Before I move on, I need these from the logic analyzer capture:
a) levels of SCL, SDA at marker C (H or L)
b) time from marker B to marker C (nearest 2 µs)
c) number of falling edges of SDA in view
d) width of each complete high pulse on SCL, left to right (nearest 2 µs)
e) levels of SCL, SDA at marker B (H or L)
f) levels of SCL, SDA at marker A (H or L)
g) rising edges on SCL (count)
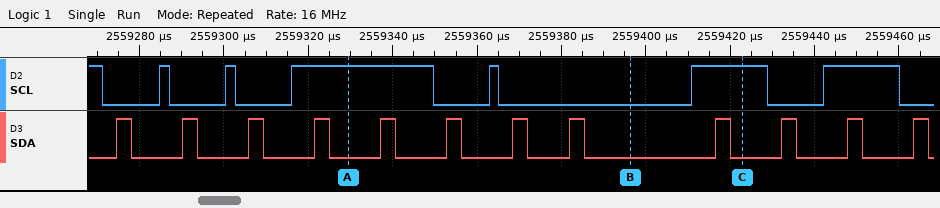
SCL=H, SDA=L
26 µs
12
2 µs, 2 µs, 34 µs, 2 µs, 18 µs, 18 µs
SCL=L, SDA=L
SCL=H, SDA=L
6
